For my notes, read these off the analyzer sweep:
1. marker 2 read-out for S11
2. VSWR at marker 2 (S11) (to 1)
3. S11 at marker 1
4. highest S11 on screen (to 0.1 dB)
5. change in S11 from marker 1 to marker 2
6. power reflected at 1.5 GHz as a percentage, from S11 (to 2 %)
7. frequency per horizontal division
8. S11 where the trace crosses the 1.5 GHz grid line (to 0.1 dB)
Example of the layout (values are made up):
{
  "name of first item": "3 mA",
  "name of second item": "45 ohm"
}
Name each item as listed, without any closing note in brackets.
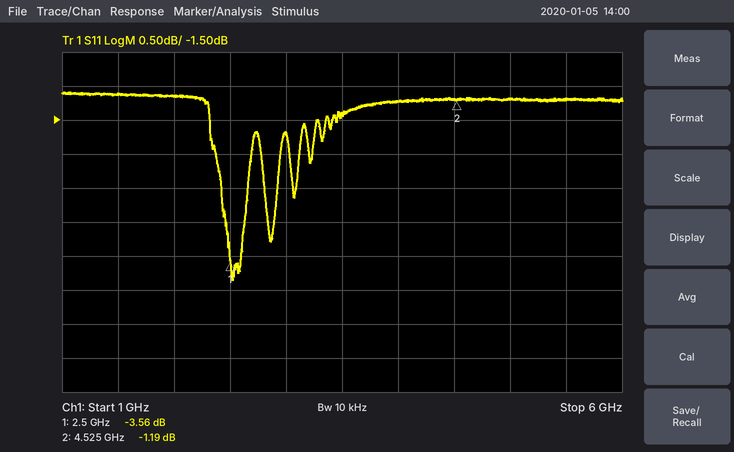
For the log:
{
  "marker 2 read-out for S11": "-1.19 dB",
  "VSWR at marker 2 (S11)": "15",
  "S11 at marker 1": "-3.56 dB",
  "highest S11 on screen": "-1.1 dB",
  "change in S11 from marker 1 to marker 2": "2.37 dB",
  "power reflected at 1.5 GHz as a percentage, from S11": "78 %",
  "frequency per horizontal division": "500 MHz",
  "S11 where the trace crosses the 1.5 GHz grid line": "-1.1 dB"
}
